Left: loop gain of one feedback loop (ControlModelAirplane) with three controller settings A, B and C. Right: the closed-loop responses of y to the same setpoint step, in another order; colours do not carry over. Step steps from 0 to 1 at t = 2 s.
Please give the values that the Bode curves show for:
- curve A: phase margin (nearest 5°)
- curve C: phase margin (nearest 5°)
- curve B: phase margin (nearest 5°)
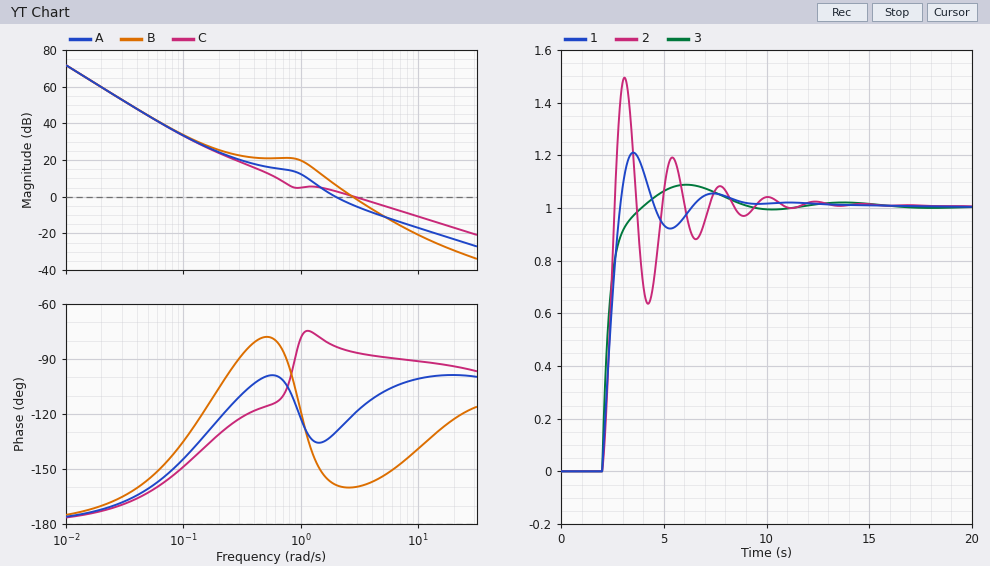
50°
95°
20°
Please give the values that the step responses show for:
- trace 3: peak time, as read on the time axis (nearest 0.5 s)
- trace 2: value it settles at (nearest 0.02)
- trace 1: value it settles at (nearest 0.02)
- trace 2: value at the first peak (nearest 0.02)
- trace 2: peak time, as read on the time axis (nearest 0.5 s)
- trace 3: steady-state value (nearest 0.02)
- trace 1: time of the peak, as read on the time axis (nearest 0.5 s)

6.0 s
1.00
1.00
1.50
3.0 s
1.00
3.5 s
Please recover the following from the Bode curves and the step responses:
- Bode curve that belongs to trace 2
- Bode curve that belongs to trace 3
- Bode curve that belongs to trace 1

B
C
A
